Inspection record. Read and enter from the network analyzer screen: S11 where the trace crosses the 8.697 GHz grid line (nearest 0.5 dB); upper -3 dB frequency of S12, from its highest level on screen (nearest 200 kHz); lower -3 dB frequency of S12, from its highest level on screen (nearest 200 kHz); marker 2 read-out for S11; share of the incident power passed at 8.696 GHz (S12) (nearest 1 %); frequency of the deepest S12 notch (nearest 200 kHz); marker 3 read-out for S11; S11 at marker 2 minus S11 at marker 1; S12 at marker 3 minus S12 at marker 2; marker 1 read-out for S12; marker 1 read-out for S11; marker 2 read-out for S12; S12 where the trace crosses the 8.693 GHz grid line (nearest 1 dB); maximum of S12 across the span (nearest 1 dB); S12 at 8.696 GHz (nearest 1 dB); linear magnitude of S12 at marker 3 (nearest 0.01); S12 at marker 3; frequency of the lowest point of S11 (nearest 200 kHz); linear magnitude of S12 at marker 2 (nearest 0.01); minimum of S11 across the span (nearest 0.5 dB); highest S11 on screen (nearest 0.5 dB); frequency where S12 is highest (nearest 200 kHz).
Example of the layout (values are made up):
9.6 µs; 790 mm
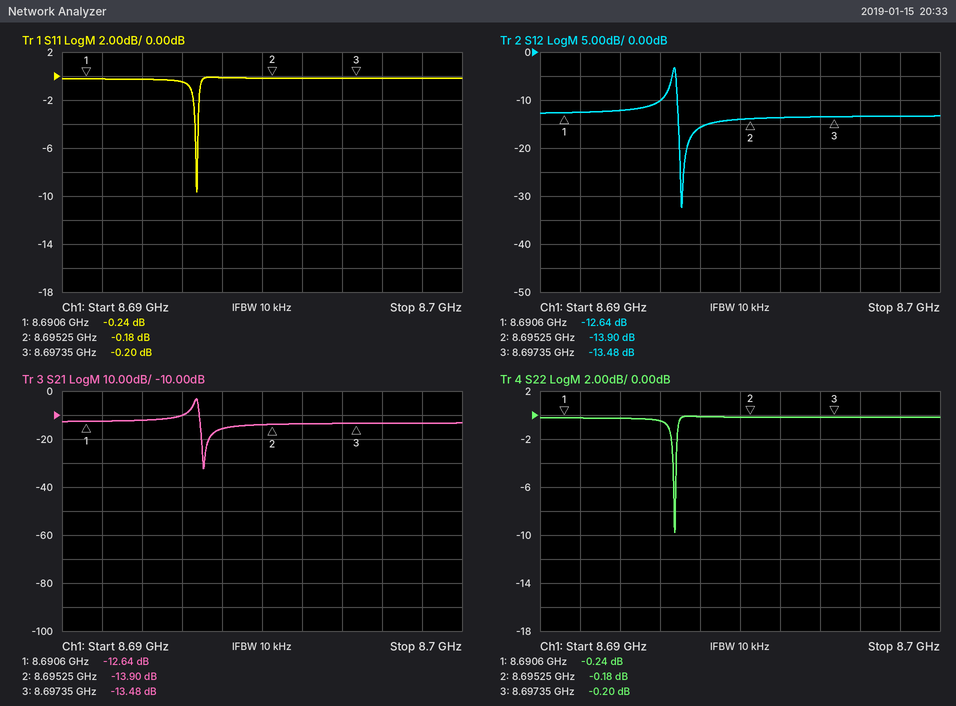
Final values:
0.0 dB; 8.6934 GHz; 8.6932 GHz; -0.18 dB; 4 %; 8.6936 GHz; -0.20 dB; 0.06 dB; 0.42 dB; -12.64 dB; -0.24 dB; -13.90 dB; -10 dB; -3 dB; -14 dB; 0.21; -13.48 dB; 8.6934 GHz; 0.20; -9.5 dB; 0.0 dB; 8.6934 GHz
